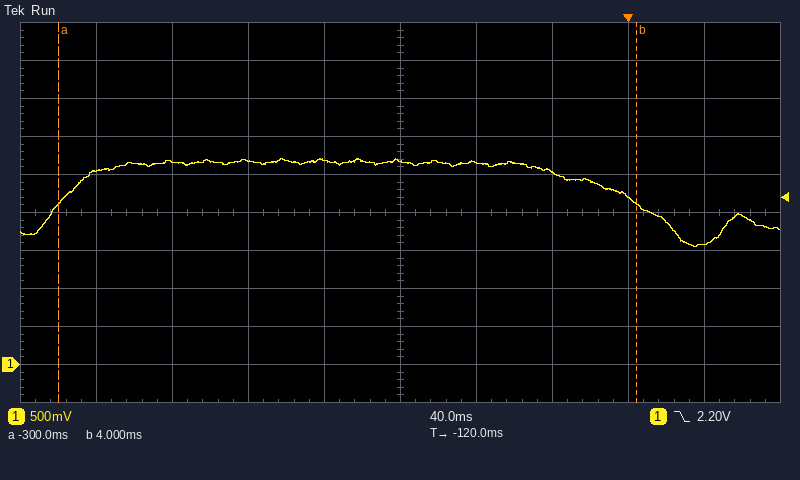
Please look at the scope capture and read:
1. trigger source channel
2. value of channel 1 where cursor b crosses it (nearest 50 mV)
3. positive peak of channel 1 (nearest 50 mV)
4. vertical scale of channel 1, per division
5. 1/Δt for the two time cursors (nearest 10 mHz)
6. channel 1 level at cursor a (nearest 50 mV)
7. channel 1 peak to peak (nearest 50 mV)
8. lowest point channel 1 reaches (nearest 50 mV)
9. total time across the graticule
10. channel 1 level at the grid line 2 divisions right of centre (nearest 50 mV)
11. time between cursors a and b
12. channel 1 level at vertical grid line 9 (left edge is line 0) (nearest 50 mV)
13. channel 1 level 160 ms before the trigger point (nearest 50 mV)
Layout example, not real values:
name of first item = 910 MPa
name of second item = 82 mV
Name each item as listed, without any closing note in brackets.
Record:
trigger source channel = channel 1
value of channel 1 where cursor b crosses it = 2.10 V
positive peak of channel 1 = 2.70 V
vertical scale of channel 1, per division = 500 mV
1/Δt for the two time cursors = 3.29 Hz
channel 1 level at cursor a = 2.10 V
channel 1 peak to peak = 1.15 V
lowest point channel 1 reaches = 1.55 V
total time across the graticule = 400 ms
channel 1 level at the grid line 2 divisions right of centre = 2.55 V
time between cursors a and b = 304 ms
channel 1 level at vertical grid line 9 (left edge is line 0) = 1.60 V
channel 1 level 160 ms before the trigger point = 2.70 V
